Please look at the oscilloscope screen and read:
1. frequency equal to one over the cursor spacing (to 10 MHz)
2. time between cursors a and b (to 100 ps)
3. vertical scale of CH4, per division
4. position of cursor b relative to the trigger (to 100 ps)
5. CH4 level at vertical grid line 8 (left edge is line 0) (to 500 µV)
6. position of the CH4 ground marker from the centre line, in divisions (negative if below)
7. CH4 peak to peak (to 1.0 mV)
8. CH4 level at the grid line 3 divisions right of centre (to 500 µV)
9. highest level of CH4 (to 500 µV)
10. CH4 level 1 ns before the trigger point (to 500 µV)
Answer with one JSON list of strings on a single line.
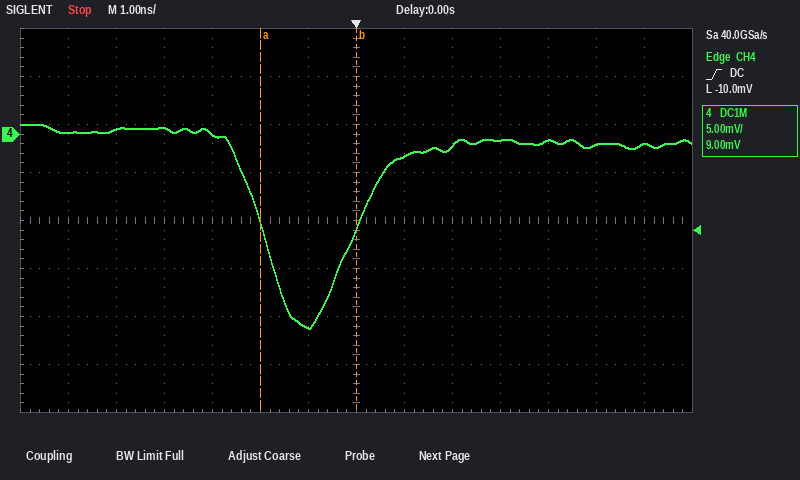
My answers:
["500 MHz", "2.0 ns", "5 mV", "0.0 ns", "-2.5 mV", "+1.8 div", "21.0 mV", "-500 µV", "1.0 mV", "-20.0 mV"]
